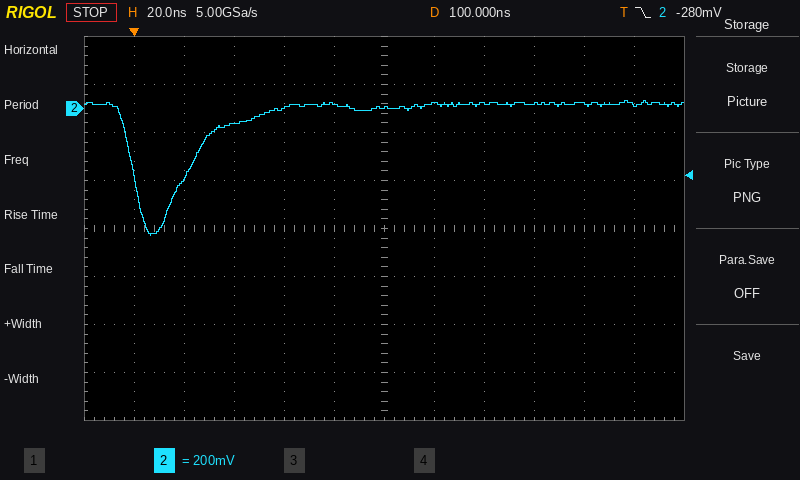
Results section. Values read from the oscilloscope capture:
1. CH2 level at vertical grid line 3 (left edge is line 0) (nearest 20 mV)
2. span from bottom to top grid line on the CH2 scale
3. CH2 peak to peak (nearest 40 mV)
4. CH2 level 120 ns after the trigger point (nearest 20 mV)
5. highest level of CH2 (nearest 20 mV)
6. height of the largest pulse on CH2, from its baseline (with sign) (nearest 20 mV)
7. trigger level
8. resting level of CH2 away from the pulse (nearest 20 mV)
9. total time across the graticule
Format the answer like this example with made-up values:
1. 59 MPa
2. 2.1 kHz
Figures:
1. -60 mV
2. 1.6 V
3. 560 mV
4. 20 mV
5. 40 mV
6. -540 mV
7. -280 mV
8. 20 mV
9. 240 ns
